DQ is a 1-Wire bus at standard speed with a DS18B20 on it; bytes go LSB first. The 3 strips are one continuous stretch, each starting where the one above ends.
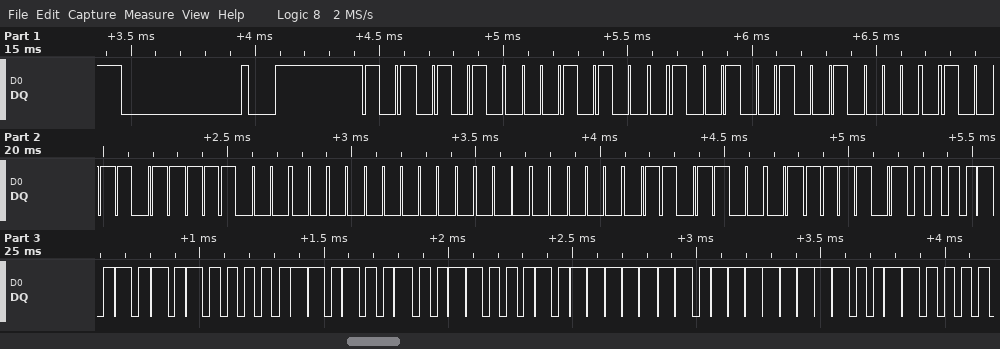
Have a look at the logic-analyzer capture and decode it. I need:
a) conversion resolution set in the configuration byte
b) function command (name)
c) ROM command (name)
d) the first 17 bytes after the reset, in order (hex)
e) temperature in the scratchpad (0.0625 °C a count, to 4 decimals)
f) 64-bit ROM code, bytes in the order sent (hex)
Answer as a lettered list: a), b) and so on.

a) 12 bits
b) Read Scratchpad
c) Match ROM
d) 55 28 92 04 D9 07 00 00 36 BE 50 05 4B 46 7F FF 0C
e) 85.0000 °C
f) 28 92 04 D9 07 00 00 36
